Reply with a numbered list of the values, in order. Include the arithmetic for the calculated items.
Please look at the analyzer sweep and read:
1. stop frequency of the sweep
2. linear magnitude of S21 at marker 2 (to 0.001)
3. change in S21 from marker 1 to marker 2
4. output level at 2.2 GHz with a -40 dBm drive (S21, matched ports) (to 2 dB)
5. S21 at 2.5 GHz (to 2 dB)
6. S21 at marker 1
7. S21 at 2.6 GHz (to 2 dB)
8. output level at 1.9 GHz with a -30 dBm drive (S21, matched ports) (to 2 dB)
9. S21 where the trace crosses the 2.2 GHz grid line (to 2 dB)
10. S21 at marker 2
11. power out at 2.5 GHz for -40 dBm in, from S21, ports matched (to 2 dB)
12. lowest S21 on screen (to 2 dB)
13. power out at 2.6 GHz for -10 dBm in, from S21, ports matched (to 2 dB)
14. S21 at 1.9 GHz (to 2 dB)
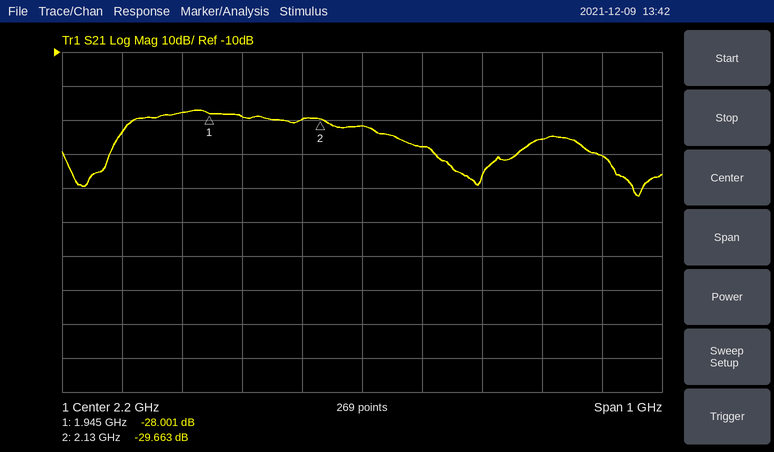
1. 2.7 GHz
2. 10^(-29.663/20) ≈ 0.033
3. -29.663 − (-28.001) = -1.662 dB
4. -40 dBm + (-32 dB) = -72 dBm
5. -36 dB
6. -28.001 dB
7. -40 dB
8. -30 dBm + (-28 dB) = -58 dBm
9. -32 dB
10. -29.663 dB
11. -40 dBm + (-36 dB) = -76 dBm
12. -52 dB
13. -10 dBm + (-40 dB) = -50 dBm
14. -28 dB
